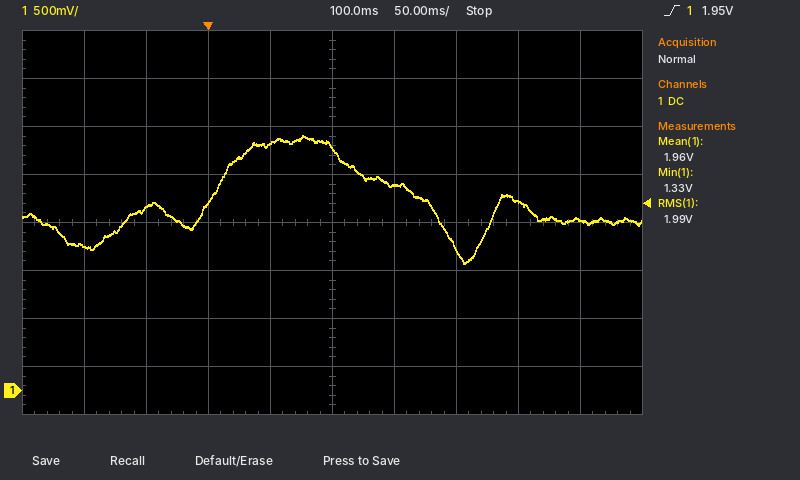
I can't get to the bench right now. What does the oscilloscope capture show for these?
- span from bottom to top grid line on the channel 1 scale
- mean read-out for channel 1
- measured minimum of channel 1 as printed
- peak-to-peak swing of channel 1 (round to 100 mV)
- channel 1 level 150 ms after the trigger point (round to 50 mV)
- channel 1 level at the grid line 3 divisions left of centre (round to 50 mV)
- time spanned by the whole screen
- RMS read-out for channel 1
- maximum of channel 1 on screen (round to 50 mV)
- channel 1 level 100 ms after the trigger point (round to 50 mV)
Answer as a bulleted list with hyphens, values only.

- 4 V
- 1.96 V
- 1.33 V
- 1.30 V
- 2.15 V
- 1.90 V
- 500 ms
- 1.99 V
- 2.65 V
- 2.55 V
